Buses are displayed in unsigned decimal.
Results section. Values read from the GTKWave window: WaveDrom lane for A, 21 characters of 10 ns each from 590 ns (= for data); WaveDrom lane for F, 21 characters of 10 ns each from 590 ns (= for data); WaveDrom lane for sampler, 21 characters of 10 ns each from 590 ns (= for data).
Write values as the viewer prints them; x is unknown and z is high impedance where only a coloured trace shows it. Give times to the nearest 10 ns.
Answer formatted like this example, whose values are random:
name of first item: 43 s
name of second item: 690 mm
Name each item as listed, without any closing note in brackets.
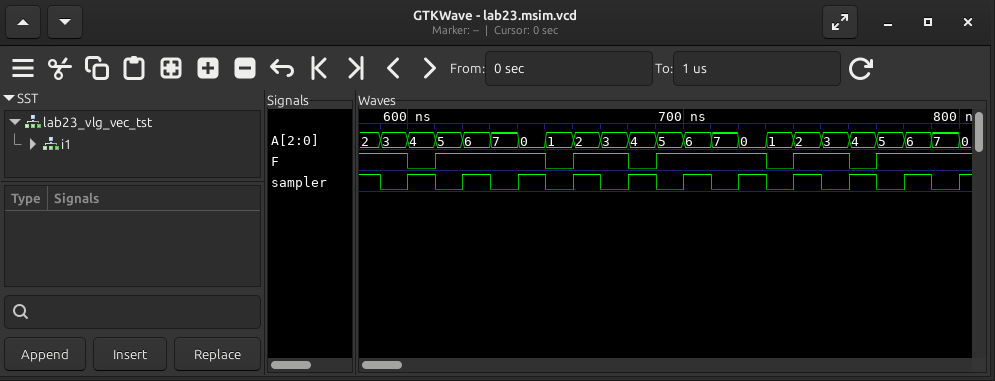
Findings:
WaveDrom lane for A, 21 characters of 10 ns each from 590 ns: {name: 'A', wave: '=====================', data: '3 4 5 6 7 0 1 2 3 4 5 6 7 0 1 2 3 4 5 6 7'}
WaveDrom lane for F, 21 characters of 10 ns each from 590 ns: {name: 'F', wave: '101...01.01...01.01..'}
WaveDrom lane for sampler, 21 characters of 10 ns each from 590 ns: {name: 'sampler', wave: '010101010101010101010'}
